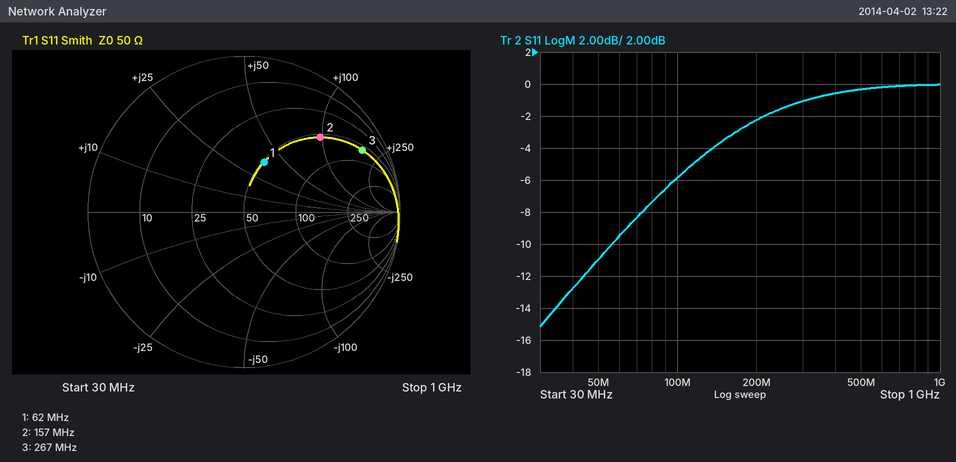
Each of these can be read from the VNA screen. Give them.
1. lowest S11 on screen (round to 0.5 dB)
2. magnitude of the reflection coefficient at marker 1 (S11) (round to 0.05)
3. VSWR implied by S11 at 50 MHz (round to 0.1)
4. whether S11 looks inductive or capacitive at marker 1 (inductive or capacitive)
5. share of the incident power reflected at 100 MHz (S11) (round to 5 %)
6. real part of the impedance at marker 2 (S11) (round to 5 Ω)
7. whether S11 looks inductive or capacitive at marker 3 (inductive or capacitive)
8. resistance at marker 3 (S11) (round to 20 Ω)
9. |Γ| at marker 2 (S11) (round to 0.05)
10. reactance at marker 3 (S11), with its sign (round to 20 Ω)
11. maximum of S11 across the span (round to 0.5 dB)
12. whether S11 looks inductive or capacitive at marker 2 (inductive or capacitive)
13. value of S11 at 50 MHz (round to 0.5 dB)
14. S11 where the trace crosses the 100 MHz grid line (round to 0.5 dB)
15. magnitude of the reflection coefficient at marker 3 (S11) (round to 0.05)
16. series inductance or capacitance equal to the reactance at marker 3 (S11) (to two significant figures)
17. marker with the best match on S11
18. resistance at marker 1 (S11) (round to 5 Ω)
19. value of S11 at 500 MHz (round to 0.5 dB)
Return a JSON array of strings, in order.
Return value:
["-15.0 dB", "0.35", "1.8", "inductive", "25 %", "55 Ω", "inductive", "60 Ω", "0.70", "+180 Ω", "0.0 dB", "inductive", "-11.0 dB", "-6.0 dB", "0.85", "110 nH", "marker 1", "50 Ω", "-0.5 dB"]
